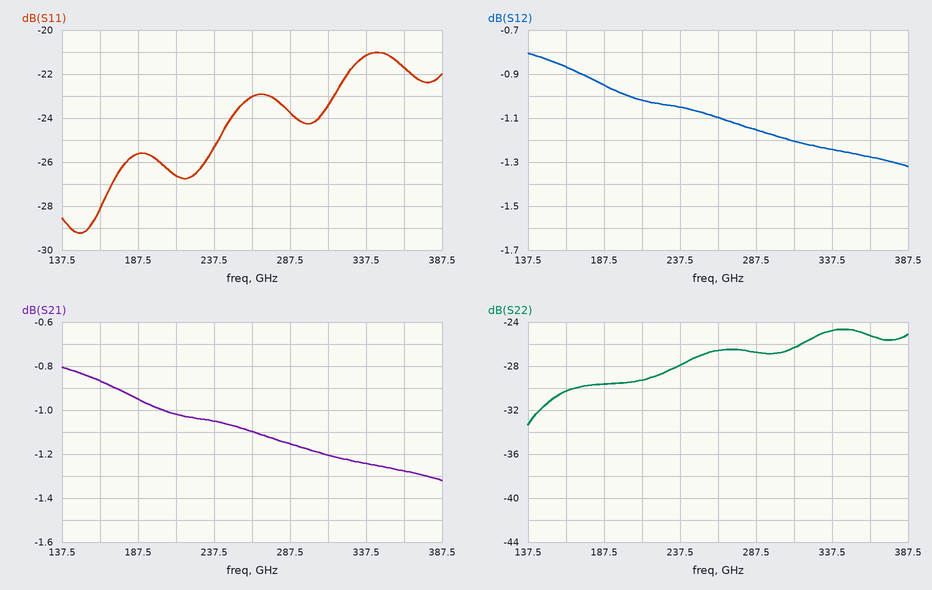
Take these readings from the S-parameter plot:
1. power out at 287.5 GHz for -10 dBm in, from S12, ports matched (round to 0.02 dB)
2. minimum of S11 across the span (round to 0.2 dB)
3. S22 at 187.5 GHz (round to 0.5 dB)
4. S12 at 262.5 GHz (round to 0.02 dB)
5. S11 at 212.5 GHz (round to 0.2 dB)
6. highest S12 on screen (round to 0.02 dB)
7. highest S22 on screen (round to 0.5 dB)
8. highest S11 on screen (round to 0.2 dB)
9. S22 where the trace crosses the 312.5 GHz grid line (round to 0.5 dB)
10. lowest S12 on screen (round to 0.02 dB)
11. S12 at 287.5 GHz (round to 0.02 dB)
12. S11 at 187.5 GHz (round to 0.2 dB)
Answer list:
-11.16 dBm
-29.2 dB
-29.5 dB
-1.10 dB
-26.6 dB
-0.80 dB
-24.5 dB
-21.0 dB
-26.5 dB
-1.32 dB
-1.16 dB
-25.6 dB
